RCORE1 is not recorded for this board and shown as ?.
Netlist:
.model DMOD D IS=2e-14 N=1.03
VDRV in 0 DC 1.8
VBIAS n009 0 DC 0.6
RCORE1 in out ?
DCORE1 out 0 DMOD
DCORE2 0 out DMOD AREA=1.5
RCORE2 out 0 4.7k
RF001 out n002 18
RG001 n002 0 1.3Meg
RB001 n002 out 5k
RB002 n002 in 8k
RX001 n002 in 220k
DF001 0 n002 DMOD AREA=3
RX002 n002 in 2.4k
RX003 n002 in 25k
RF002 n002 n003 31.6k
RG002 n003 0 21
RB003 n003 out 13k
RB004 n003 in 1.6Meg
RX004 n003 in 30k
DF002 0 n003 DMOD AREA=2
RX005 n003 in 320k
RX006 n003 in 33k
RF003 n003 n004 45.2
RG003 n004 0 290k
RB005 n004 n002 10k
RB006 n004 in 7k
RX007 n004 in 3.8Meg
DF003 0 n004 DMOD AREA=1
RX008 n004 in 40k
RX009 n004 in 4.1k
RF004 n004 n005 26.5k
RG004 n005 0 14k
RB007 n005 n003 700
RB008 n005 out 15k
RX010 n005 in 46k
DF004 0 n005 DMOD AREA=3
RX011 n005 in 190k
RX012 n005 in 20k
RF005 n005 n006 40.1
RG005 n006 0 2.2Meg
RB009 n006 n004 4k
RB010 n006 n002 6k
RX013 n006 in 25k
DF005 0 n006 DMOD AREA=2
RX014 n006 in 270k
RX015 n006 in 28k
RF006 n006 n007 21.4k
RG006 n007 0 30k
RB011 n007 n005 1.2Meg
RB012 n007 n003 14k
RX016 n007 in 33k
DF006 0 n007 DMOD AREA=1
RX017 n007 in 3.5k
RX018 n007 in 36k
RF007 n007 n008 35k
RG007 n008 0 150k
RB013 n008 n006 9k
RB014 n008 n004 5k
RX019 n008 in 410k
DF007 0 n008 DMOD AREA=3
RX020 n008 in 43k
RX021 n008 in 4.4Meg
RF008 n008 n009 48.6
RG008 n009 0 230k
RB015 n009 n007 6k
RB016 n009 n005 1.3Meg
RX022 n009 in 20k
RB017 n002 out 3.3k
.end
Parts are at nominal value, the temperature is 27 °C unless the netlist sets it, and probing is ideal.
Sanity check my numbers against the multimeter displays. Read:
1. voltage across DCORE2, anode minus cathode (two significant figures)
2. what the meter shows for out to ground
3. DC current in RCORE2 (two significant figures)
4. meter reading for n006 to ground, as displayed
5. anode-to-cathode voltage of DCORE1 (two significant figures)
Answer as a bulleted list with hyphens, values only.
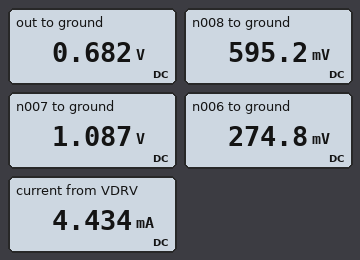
- -680 mV
- 0.682 V
- 150 µA
- 274.8 mV
- 680 mV
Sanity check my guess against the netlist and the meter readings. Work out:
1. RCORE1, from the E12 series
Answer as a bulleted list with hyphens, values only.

- 470 Ω
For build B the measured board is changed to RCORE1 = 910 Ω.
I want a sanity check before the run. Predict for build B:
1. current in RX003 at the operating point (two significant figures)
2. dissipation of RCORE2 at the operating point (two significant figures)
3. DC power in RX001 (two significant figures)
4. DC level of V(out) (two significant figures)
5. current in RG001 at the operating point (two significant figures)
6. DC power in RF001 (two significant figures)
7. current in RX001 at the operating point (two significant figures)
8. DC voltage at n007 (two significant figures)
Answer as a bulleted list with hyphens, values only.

- 45 µA
- 95 µW
- 5.7 µW
- 670 mV
- 520 nA
- 4.6 µW
- 5.1 µA
- 1.1 V
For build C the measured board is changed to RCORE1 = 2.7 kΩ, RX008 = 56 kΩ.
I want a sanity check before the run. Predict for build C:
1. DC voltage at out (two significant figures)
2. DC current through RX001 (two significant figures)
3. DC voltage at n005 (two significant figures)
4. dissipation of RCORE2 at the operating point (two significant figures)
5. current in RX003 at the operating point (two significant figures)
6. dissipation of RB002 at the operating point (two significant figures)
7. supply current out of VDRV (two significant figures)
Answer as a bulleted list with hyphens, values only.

- 650 mV
- 5.2 µA
- 260 mV
- 89 µW
- 46 µA
- 160 µW
- 2.5 mA
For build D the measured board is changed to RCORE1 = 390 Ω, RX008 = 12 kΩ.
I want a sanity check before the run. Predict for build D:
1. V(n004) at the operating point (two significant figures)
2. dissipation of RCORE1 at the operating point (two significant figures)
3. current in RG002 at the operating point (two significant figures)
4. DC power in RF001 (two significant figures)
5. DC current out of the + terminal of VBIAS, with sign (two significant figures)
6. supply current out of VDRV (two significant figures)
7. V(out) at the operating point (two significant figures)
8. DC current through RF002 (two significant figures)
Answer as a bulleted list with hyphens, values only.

- 81 mV
- 3.2 mW
- 1.6 mA
- 4.3 µW
- -41 µA
- 5.0 mA
- 690 mV
- 21 µA
